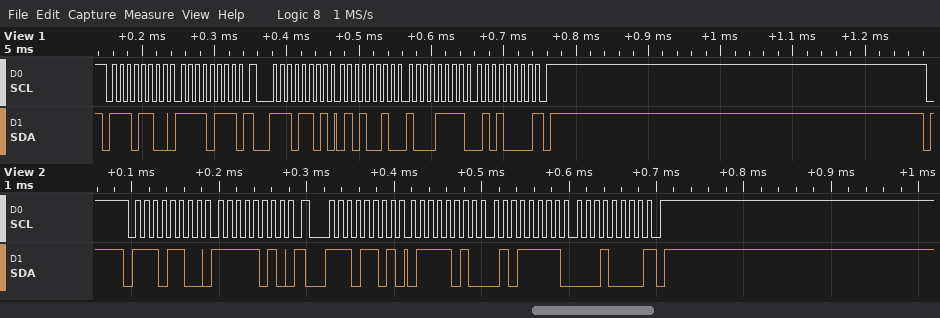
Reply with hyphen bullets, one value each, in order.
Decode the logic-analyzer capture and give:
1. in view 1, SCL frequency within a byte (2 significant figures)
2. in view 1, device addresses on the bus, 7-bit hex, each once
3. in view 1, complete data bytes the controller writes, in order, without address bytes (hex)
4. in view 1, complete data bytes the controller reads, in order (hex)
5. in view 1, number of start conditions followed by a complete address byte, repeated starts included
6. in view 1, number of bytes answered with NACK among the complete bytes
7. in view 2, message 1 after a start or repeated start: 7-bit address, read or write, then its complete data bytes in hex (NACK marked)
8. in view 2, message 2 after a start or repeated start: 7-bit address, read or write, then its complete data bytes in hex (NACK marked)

- 100 kHz
- 0x76
- F7
- 52 8F 50
- 2
- 1
- 0x76 write: FA
- 0x76 read: 7A 5F 10 NACK
